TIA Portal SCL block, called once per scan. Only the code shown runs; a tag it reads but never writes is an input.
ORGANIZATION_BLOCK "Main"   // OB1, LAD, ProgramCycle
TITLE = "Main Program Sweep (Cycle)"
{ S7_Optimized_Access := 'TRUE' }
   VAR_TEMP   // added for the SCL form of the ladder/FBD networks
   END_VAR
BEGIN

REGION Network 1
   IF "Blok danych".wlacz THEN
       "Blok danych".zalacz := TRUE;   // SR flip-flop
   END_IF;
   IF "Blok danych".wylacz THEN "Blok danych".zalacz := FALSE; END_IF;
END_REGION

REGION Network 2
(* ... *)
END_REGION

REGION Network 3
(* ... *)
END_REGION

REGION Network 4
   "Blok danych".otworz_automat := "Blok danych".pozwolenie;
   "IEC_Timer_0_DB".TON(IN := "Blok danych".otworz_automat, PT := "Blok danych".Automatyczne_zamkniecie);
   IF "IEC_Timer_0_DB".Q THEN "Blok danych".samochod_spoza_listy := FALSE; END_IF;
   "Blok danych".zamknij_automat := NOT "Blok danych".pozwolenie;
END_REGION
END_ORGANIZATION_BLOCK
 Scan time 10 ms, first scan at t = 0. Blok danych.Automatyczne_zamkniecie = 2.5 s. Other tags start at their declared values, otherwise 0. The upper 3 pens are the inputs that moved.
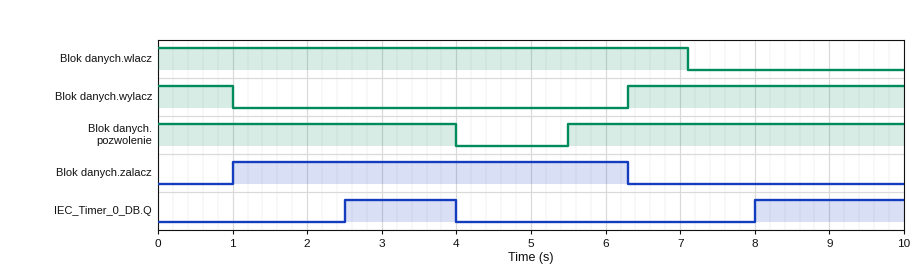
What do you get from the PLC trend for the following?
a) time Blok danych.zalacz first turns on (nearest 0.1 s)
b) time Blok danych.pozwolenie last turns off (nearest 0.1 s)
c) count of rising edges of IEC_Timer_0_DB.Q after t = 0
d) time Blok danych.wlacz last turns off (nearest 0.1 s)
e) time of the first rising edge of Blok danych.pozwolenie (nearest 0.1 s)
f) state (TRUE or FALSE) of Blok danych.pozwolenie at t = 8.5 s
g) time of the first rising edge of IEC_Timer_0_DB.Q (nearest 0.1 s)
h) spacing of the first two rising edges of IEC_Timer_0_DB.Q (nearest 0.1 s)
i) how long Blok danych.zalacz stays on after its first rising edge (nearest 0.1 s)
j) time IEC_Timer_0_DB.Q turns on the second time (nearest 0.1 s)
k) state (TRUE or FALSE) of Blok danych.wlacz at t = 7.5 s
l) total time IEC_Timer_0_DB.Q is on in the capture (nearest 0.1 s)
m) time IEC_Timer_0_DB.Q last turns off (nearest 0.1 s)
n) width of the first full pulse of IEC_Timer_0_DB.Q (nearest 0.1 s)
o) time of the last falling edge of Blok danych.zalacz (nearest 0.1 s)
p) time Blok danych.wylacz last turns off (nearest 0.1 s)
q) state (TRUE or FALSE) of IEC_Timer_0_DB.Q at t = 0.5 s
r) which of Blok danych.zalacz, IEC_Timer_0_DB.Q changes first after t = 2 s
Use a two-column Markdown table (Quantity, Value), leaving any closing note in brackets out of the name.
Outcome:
| Quantity | Value |
|---|---|
| time Blok danych.zalacz first turns on | 1.0 s |
| time Blok danych.pozwolenie last turns off | 4.0 s |
| count of rising edges of IEC_Timer_0_DB.Q after t = 0 | 2 |
| time Blok danych.wlacz last turns off | 7.1 s |
| time of the first rising edge of Blok danych.pozwolenie | 5.5 s |
| state (TRUE or FALSE) of Blok danych.pozwolenie at t = 8.5 s | TRUE |
| time of the first rising edge of IEC_Timer_0_DB.Q | 2.5 s |
| spacing of the first two rising edges of IEC_Timer_0_DB.Q | 5.5 s |
| how long Blok danych.zalacz stays on after its first rising edge | 5.3 s |
| time IEC_Timer_0_DB.Q turns on the second time | 8.0 s |
| state (TRUE or FALSE) of Blok danych.wlacz at t = 7.5 s | FALSE |
| total time IEC_Timer_0_DB.Q is on in the capture | 3.5 s |
| time IEC_Timer_0_DB.Q last turns off | 4.0 s |
| width of the first full pulse of IEC_Timer_0_DB.Q | 1.5 s |
| time of the last falling edge of Blok danych.zalacz | 6.3 s |
| time Blok danych.wylacz last turns off | 1.0 s |
| state (TRUE or FALSE) of IEC_Timer_0_DB.Q at t = 0.5 s | FALSE |
| which of Blok danych.zalacz, IEC_Timer_0_DB.Q changes first after t = 2 s | IEC_Timer_0_DB.Q |
